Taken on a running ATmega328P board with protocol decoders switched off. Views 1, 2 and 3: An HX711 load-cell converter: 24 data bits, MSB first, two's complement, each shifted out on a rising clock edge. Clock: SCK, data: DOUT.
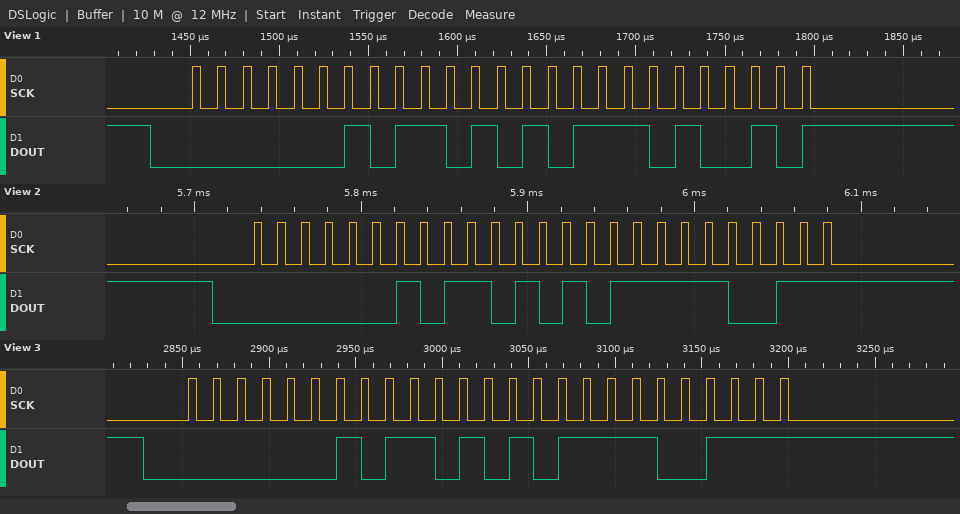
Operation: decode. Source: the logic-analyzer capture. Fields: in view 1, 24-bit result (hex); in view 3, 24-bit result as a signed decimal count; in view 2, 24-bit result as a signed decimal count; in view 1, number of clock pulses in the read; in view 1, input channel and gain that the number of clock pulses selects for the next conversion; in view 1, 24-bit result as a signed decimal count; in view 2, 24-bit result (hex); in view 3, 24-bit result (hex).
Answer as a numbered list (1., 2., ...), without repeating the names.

1. 0x02D5D2
2. 185831
3. 185843
4. 25
5. channel A, gain 128
6. 185810
7. 0x02D5F3
8. 0x02D5E7
